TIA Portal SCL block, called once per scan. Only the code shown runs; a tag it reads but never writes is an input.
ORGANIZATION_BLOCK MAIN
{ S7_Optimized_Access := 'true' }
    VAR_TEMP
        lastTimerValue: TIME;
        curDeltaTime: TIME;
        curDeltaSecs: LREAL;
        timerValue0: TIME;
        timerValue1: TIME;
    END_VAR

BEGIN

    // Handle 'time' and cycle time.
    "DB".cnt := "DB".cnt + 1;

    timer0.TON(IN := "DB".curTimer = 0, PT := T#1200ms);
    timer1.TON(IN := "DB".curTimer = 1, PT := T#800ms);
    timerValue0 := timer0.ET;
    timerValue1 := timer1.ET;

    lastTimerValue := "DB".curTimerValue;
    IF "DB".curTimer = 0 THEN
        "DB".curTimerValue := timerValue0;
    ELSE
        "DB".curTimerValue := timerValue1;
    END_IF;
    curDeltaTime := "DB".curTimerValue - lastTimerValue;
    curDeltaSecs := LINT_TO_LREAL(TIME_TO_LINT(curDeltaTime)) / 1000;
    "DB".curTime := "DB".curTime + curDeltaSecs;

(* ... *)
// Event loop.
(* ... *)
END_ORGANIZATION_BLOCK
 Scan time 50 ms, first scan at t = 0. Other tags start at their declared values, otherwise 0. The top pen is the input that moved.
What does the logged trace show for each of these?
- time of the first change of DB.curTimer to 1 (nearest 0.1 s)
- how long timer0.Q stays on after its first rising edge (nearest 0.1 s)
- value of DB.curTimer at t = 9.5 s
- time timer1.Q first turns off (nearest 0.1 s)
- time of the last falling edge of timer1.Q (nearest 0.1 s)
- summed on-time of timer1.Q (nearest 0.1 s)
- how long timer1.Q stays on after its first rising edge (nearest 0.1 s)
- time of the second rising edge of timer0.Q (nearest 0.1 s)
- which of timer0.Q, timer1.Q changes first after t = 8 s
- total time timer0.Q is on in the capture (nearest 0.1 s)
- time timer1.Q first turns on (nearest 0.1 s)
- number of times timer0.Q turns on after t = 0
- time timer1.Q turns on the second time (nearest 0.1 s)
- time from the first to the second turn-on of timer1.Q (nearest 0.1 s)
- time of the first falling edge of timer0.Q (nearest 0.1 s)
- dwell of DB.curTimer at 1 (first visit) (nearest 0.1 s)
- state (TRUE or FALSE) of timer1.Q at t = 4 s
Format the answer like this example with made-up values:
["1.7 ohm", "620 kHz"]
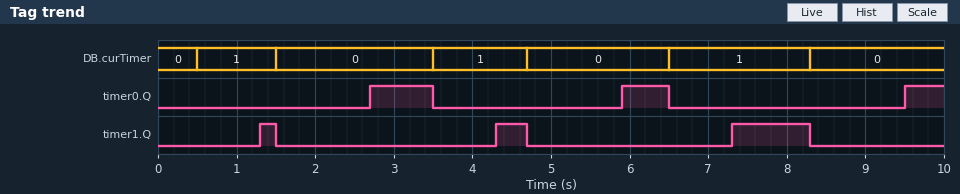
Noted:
["0.5 s", "0.8 s", "0", "1.5 s", "8.3 s", "1.6 s", "0.2 s", "5.9 s", "timer1.Q", "1.9 s", "1.3 s", "3", "4.3 s", "3.0 s", "3.5 s", "1.0 s", "FALSE"]
